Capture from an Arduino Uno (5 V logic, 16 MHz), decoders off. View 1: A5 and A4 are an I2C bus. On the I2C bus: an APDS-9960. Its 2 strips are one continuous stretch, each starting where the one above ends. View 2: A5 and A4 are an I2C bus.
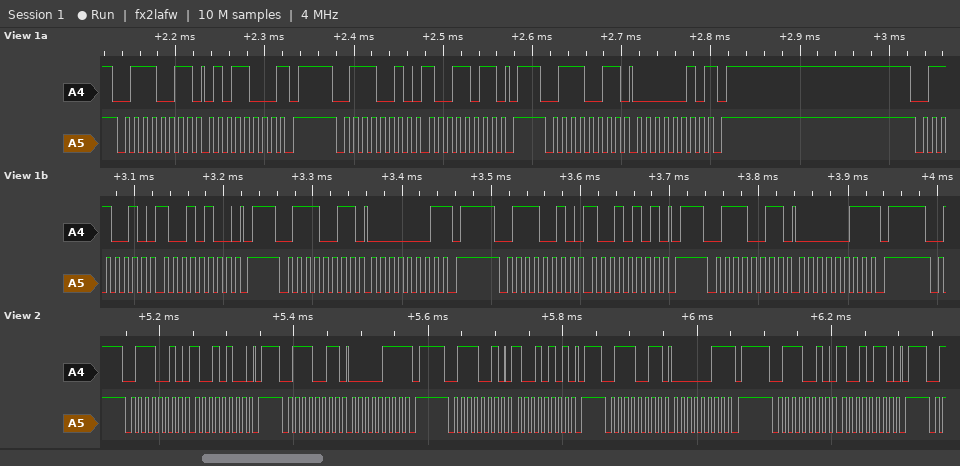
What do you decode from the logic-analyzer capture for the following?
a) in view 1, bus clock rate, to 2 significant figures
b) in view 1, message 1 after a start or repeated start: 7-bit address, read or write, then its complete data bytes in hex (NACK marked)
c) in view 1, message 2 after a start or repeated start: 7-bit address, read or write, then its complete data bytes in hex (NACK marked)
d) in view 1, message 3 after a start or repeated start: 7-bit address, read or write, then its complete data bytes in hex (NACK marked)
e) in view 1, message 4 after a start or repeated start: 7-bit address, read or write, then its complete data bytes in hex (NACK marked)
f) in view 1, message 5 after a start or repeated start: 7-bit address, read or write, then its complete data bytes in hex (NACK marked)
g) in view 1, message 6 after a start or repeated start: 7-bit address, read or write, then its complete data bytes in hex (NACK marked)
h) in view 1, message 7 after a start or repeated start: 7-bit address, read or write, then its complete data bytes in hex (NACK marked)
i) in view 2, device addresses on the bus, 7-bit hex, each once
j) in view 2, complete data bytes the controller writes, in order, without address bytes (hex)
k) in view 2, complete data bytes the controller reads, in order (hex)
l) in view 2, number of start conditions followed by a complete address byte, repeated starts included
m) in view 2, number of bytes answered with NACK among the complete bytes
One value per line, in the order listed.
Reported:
100 kHz
0x39 read: 58 NACK
0x39 write: 9B
0x39 read: 02 NACK
0x39 write: 94
0x39 read: 01 NACK
0x39 write: 95
0x39 read: 03 NACK
0x39
94 95 96
07 03
5
2
